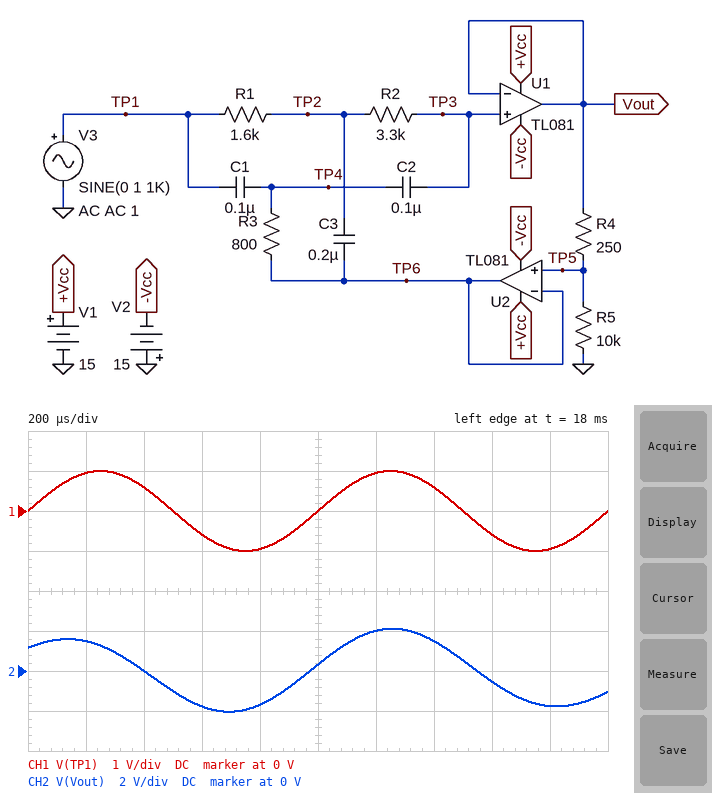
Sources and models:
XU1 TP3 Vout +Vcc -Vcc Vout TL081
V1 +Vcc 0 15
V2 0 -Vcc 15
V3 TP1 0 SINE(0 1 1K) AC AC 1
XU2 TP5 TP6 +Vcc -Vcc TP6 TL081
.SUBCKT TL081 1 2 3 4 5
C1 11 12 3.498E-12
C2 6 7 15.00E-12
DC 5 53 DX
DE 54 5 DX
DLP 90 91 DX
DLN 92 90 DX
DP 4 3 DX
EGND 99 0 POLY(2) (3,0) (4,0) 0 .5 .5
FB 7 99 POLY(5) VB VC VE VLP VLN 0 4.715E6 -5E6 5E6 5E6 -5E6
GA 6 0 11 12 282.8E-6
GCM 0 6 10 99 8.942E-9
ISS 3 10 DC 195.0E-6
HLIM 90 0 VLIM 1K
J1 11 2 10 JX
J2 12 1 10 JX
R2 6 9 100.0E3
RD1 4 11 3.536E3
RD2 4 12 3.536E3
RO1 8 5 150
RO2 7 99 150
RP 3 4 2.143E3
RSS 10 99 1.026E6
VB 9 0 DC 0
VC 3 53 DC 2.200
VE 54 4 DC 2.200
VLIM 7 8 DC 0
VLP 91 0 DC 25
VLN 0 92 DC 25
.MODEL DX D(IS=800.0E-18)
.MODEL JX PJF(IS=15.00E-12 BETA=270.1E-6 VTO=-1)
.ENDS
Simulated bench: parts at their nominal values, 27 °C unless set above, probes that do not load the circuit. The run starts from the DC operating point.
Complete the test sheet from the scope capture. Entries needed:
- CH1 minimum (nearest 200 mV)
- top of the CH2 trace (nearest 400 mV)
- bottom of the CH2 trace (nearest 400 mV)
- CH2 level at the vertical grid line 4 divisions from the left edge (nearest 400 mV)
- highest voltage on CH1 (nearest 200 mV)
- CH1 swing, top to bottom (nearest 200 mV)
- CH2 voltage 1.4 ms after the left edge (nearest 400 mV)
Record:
-1.0 V
2.0 V
-2.0 V
-1.6 V
1.0 V
2.0 V
1.6 V
